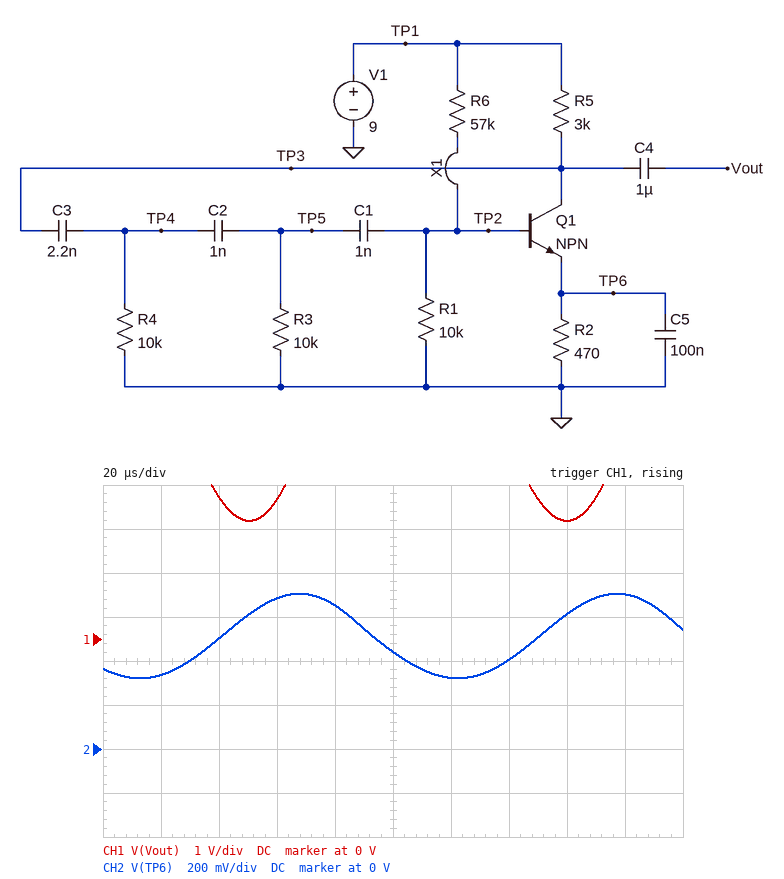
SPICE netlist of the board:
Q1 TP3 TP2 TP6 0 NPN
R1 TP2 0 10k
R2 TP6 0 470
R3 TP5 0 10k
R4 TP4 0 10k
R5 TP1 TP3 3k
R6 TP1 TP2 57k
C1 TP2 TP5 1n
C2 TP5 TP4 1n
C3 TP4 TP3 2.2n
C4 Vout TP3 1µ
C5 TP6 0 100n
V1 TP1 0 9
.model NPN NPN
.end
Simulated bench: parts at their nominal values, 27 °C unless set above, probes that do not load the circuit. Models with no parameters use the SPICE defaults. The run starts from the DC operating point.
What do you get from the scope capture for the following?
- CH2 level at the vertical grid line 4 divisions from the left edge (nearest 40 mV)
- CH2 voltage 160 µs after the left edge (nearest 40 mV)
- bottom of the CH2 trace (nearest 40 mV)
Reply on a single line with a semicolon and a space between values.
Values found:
640 mV; 600 mV; 320 mV
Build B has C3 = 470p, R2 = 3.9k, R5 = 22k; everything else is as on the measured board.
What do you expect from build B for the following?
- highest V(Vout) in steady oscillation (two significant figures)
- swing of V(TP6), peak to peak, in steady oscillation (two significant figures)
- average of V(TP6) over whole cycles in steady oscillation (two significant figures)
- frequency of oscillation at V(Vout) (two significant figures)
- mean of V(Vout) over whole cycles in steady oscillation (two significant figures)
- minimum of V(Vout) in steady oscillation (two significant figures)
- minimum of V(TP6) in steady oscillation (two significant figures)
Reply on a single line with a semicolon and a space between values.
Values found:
8.5 V; 72 mV; 620 mV; 7.8 kHz; 5.5 V; 2.1 V; 590 mV
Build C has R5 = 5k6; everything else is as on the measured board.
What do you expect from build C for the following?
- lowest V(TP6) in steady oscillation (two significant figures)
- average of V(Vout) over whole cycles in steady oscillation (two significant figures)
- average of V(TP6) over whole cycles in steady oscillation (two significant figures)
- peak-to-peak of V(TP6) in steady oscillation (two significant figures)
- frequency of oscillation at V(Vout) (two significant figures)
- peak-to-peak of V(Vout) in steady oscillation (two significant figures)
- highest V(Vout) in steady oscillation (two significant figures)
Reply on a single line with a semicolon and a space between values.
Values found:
320 mV; 3.6 V; 460 mV; 270 mV; 7.8 kHz; 6.3 V; 6.8 V
